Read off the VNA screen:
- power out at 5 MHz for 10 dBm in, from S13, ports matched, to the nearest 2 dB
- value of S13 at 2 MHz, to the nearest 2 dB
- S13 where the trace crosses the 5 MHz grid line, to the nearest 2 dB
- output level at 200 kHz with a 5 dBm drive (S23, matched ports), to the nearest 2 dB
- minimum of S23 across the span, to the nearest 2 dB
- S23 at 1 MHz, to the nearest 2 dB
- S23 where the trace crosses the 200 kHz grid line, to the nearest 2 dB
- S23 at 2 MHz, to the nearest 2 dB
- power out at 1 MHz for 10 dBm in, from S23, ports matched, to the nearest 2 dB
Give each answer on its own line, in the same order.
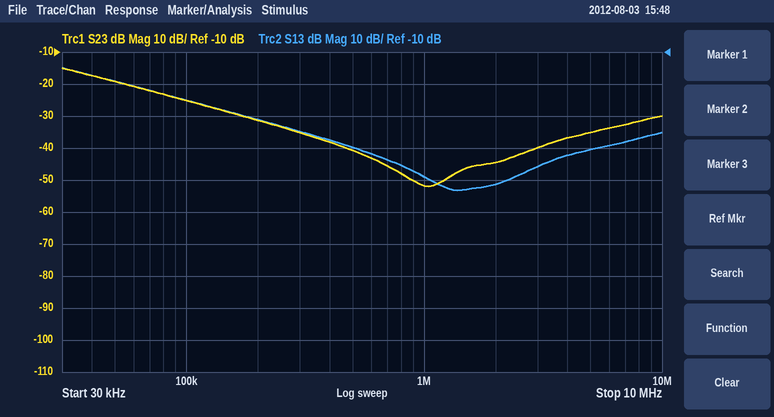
-30 dBm
-52 dB
-40 dB
-26 dBm
-52 dB
-52 dB
-32 dB
-44 dB
-42 dBm
